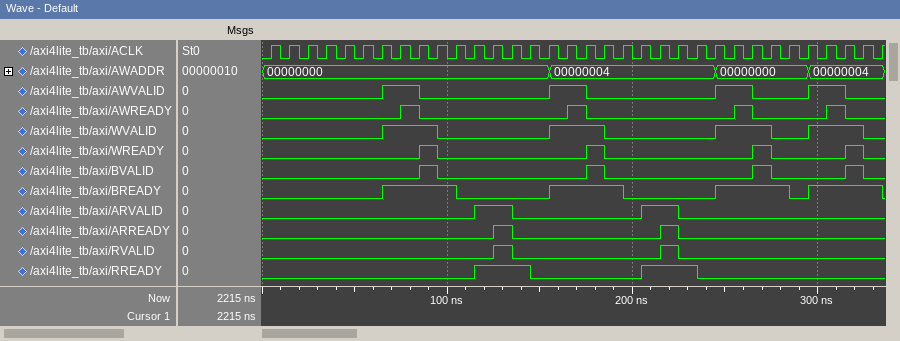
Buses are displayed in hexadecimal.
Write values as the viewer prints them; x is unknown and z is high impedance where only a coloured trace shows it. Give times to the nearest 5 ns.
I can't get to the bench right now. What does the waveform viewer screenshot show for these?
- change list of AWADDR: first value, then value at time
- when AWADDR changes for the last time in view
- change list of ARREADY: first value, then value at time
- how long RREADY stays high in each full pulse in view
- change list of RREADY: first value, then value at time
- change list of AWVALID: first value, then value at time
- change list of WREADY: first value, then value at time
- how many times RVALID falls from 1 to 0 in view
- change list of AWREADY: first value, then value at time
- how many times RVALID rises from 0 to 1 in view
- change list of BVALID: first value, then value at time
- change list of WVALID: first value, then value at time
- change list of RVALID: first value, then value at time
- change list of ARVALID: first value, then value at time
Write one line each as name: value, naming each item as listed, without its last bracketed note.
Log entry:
change list of AWADDR: first value, then value at time: 00000000, 00000004 at 155 ns, 00000000 at 245 ns, 00000004 at 295 ns
when AWADDR changes for the last time in view: 295 ns
change list of ARREADY: first value, then value at time: 0, 1 at 125 ns, 0 at 135 ns, 1 at 215 ns, 0 at 225 ns
how long RREADY stays high in each full pulse in view: 30 ns, 30 ns
change list of RREADY: first value, then value at time: 0, 1 at 115 ns, 0 at 145 ns, 1 at 205 ns, 0 at 235 ns
change list of AWVALID: first value, then value at time: 0, 1 at 65 ns, 0 at 85 ns, 1 at 155 ns, 0 at 175 ns, 1 at 245 ns, 0 at 265 ns, 1 at 295 ns, 0 at 315 ns
change list of WREADY: first value, then value at time: 0, 1 at 85 ns, 0 at 95 ns, 1 at 175 ns, 0 at 185 ns, 1 at 265 ns, 0 at 275 ns, 1 at 315 ns, 0 at 325 ns
how many times RVALID falls from 1 to 0 in view: 2
change list of AWREADY: first value, then value at time: 0, 1 at 75 ns, 0 at 85 ns, 1 at 165 ns, 0 at 175 ns, 1 at 255 ns, 0 at 265 ns, 1 at 305 ns, 0 at 315 ns
how many times RVALID rises from 0 to 1 in view: 2
change list of BVALID: first value, then value at time: 0, 1 at 85 ns, 0 at 95 ns, 1 at 175 ns, 0 at 185 ns, 1 at 265 ns, 0 at 275 ns, 1 at 315 ns, 0 at 325 ns
change list of WVALID: first value, then value at time: 0, 1 at 65 ns, 0 at 95 ns, 1 at 155 ns, 0 at 185 ns, 1 at 245 ns, 0 at 275 ns, 1 at 295 ns, 0 at 325 ns
change list of RVALID: first value, then value at time: 0, 1 at 125 ns, 0 at 135 ns, 1 at 215 ns, 0 at 225 ns
change list of ARVALID: first value, then value at time: 0, 1 at 115 ns, 0 at 135 ns, 1 at 205 ns, 0 at 225 ns
